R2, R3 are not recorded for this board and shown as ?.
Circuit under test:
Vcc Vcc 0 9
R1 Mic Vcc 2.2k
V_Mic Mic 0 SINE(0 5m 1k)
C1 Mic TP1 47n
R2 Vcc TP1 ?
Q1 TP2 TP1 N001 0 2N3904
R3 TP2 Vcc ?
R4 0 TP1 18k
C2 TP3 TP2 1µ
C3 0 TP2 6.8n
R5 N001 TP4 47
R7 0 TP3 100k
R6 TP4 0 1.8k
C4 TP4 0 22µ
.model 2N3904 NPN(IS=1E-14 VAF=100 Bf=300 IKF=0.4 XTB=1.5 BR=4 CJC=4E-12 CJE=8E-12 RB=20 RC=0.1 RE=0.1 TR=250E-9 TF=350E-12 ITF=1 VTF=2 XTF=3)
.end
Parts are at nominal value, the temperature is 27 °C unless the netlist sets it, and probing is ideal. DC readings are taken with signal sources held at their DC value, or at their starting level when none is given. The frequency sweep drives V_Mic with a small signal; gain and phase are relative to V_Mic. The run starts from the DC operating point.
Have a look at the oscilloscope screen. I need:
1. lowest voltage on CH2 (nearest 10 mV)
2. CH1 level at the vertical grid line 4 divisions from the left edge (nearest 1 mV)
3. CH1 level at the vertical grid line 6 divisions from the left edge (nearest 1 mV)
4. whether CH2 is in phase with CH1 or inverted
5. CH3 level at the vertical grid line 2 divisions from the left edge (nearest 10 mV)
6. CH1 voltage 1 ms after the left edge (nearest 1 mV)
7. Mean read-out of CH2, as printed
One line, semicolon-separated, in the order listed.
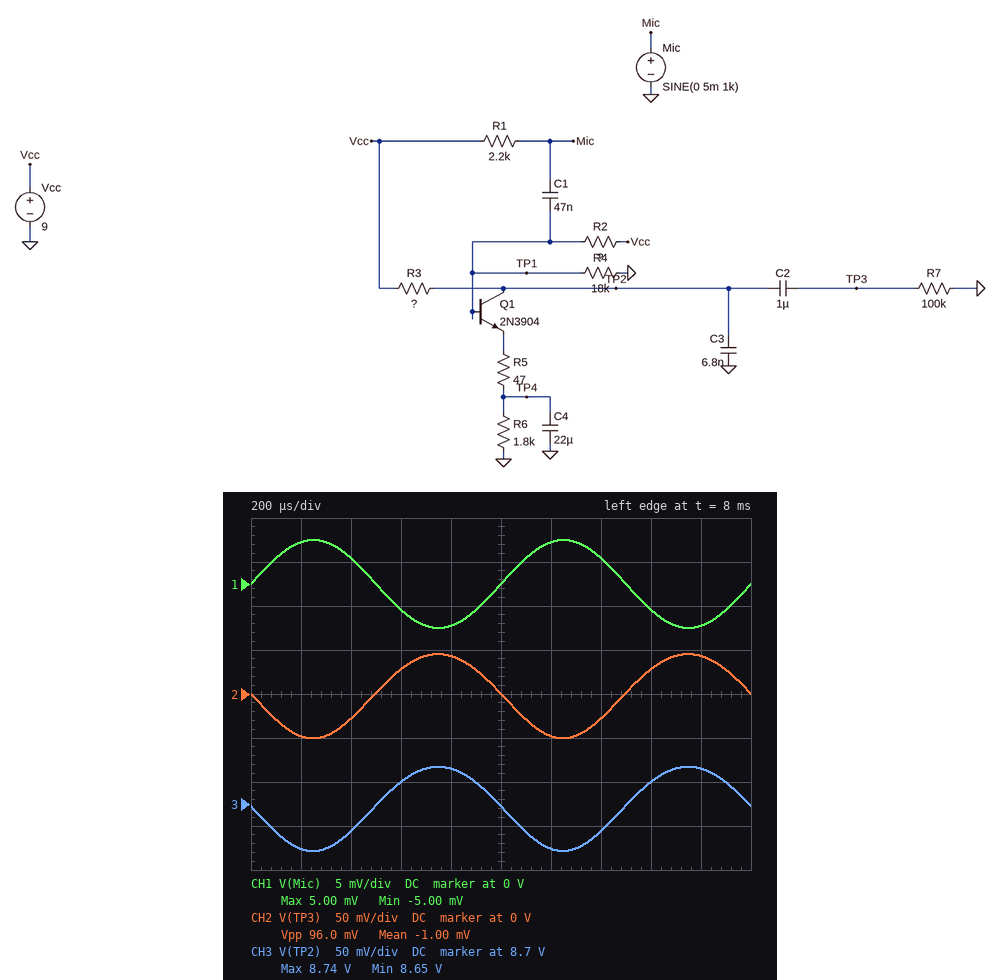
-50 mV; -5 mV; 5 mV; inverted; 8.67 V; 0 V; -1.00 mV
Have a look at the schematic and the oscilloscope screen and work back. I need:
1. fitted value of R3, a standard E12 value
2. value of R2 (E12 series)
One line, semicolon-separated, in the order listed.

5.6 kΩ; 220 kΩ
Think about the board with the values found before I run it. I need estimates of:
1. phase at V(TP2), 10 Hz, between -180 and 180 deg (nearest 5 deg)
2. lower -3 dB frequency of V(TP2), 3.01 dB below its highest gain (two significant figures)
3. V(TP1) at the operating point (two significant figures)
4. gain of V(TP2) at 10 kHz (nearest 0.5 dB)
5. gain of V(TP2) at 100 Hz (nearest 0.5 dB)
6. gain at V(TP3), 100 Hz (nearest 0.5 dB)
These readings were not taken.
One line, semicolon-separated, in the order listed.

-55 deg; 210 Hz; 680 mV; 12.0 dB; 12.0 dB; 12.0 dB
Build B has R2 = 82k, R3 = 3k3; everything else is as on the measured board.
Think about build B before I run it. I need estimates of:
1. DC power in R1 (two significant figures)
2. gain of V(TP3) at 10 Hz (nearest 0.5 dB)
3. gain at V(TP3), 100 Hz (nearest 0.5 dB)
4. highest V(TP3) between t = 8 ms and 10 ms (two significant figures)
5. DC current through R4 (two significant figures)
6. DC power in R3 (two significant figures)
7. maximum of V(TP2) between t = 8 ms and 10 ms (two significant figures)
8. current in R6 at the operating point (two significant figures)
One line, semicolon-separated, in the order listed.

37 mW; -14.5 dB; 17.5 dB; 150 mV; 89 µA; 880 µW; 7.4 V; 520 µA
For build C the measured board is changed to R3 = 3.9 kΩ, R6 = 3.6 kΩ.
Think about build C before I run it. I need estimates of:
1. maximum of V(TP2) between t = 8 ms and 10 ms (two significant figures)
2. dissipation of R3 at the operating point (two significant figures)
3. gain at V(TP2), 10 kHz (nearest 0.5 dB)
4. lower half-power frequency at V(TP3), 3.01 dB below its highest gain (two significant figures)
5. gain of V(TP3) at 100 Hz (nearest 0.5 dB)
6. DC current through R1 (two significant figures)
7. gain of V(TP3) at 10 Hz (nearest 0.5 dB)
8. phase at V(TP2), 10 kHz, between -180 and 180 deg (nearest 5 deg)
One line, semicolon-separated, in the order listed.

8.9 V; 3.9 µW; 7.0 dB; 200 Hz; 5.0 dB; 4.1 mA; -17.0 dB; 125 deg
